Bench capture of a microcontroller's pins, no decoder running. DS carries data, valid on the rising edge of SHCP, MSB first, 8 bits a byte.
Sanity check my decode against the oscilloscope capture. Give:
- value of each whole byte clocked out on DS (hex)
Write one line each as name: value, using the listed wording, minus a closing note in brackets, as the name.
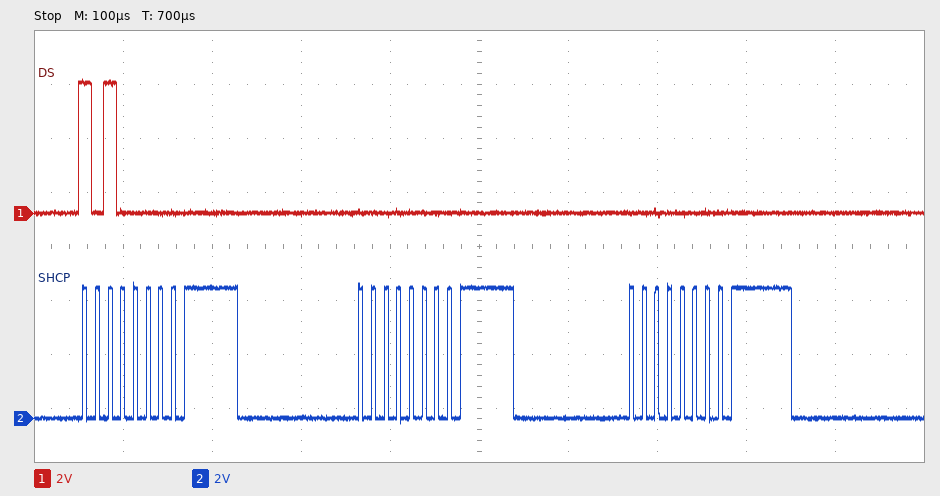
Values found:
value of each whole byte clocked out on DS: A0 00 00
